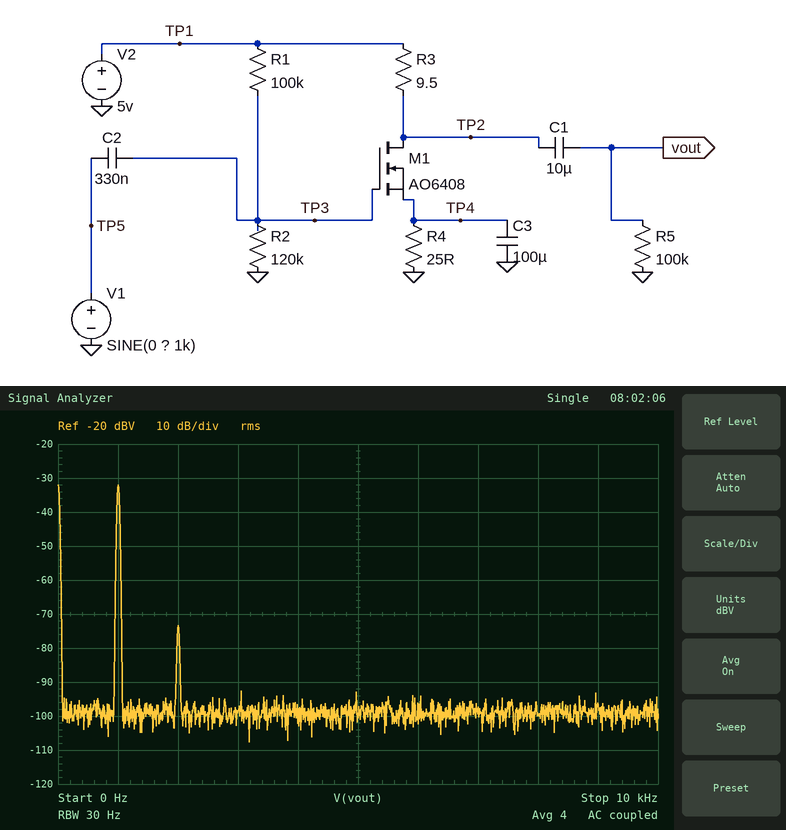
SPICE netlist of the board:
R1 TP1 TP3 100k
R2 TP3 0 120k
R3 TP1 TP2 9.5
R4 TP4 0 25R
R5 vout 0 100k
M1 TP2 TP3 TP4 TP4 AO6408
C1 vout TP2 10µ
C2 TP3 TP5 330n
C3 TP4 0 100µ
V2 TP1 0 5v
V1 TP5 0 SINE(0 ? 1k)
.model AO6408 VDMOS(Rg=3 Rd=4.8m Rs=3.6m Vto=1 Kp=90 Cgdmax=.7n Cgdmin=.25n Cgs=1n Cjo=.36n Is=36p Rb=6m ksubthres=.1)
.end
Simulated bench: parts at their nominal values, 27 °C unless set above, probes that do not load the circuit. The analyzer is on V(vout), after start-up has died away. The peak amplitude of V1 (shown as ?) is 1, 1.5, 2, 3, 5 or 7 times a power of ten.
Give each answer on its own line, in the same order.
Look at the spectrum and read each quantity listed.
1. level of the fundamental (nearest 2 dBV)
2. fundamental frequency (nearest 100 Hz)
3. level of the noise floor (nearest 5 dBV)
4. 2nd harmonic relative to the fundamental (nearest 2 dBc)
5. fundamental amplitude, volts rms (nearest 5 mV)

-32 dBV
1.0 kHz
-100 dBV
-42 dBc
25 mV
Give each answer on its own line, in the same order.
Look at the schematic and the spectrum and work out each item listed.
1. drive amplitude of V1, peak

7 mV
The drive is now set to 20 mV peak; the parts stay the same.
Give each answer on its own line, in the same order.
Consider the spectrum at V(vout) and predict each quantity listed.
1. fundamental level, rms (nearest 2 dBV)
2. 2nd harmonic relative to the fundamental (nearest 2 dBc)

-22 dBV
-32 dBc
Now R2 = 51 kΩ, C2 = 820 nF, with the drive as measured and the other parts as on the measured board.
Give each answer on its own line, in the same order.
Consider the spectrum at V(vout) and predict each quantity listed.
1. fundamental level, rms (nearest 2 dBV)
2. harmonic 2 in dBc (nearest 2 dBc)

-34 dBV
-34 dBc
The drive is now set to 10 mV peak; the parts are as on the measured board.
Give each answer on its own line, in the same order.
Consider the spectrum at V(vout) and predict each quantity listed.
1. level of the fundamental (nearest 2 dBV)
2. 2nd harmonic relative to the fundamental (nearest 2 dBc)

-28 dBV
-38 dBc
